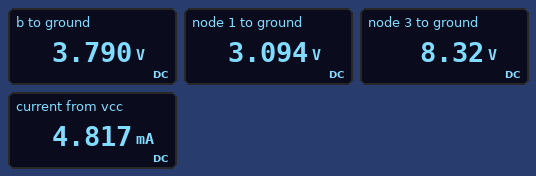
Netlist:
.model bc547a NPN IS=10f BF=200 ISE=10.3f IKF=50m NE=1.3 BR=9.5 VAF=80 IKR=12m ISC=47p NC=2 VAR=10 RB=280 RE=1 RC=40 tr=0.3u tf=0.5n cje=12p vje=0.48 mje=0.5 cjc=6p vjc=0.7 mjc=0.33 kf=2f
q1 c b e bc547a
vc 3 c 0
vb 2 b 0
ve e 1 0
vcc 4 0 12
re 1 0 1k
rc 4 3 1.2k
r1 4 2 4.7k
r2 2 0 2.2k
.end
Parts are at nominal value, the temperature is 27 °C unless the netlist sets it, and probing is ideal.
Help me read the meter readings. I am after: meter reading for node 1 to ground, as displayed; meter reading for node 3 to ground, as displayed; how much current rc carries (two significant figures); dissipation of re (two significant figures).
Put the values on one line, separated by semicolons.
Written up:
3.094 V; 8.32 V; 3.1 mA; 9.6 mW
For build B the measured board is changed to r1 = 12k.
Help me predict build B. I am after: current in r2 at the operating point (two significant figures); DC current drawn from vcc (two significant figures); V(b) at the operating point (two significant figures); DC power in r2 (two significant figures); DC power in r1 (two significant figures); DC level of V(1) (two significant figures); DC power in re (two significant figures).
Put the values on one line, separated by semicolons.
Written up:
840 µA; 2.0 mA; 1.8 V; 1.5 mW; 8.6 mW; 1.2 V; 1.4 mW
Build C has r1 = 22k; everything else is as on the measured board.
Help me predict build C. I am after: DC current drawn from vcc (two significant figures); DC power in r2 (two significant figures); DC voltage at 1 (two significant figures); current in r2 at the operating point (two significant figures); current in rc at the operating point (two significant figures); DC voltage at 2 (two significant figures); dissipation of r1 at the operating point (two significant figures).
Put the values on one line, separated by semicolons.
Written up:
940 µA; 530 µW; 450 mV; 490 µA; 450 µA; 1.1 V; 5.4 mW
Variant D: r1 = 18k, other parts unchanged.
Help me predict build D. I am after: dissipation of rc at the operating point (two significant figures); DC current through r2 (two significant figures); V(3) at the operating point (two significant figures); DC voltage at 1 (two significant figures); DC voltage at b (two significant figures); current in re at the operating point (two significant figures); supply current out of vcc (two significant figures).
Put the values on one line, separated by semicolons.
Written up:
500 µW; 590 µA; 11 V; 650 mV; 1.3 V; 650 µA; 1.2 mA
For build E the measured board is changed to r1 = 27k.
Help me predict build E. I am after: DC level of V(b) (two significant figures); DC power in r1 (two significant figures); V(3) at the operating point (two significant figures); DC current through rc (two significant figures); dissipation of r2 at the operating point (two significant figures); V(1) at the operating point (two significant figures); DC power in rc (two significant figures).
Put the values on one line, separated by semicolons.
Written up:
900 mV; 4.6 mW; 12 V; 280 µA; 370 µW; 280 mV; 91 µW
